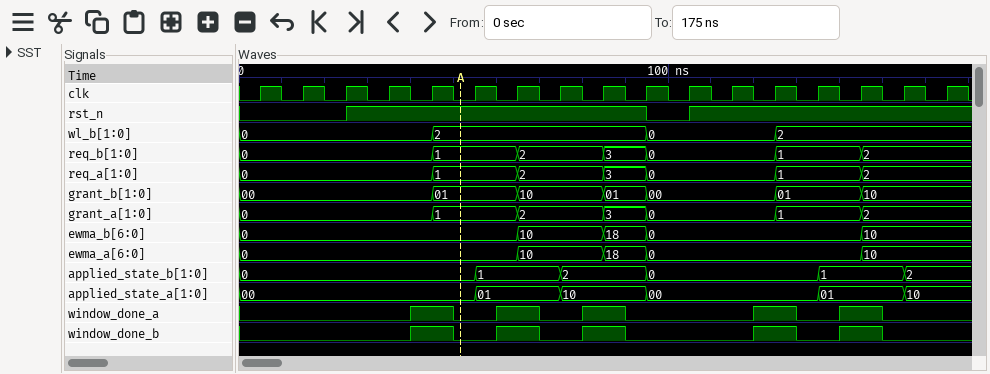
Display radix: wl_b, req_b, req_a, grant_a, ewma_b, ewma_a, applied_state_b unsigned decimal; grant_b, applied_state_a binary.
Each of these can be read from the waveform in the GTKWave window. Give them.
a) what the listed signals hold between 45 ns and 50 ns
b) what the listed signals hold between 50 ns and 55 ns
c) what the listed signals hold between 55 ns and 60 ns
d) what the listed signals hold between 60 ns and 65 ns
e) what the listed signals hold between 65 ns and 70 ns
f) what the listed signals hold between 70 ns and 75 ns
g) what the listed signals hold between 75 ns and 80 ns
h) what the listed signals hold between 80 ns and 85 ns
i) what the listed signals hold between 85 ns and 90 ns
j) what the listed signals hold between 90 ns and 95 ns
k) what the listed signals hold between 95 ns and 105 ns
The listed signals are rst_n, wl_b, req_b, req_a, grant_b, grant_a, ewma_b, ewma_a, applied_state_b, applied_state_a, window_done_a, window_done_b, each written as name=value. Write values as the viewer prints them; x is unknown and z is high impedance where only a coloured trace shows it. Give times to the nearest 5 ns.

rst_n=1, wl_b=2, req_b=1, req_a=1, grant_b=01, grant_a=1, ewma_b=0, ewma_a=0, applied_state_b=0, applied_state_a=00, window_done_a=1, window_done_b=1
rst_n=1, wl_b=2, req_b=1, req_a=1, grant_b=01, grant_a=1, ewma_b=0, ewma_a=0, applied_state_b=0, applied_state_a=00, window_done_a=0, window_done_b=0
rst_n=1, wl_b=2, req_b=1, req_a=1, grant_b=01, grant_a=1, ewma_b=0, ewma_a=0, applied_state_b=1, applied_state_a=01, window_done_a=0, window_done_b=0
rst_n=1, wl_b=2, req_b=1, req_a=1, grant_b=01, grant_a=1, ewma_b=0, ewma_a=0, applied_state_b=1, applied_state_a=01, window_done_a=1, window_done_b=1
rst_n=1, wl_b=2, req_b=2, req_a=2, grant_b=10, grant_a=2, ewma_b=10, ewma_a=10, applied_state_b=1, applied_state_a=01, window_done_a=1, window_done_b=1
rst_n=1, wl_b=2, req_b=2, req_a=2, grant_b=10, grant_a=2, ewma_b=10, ewma_a=10, applied_state_b=1, applied_state_a=01, window_done_a=0, window_done_b=0
rst_n=1, wl_b=2, req_b=2, req_a=2, grant_b=10, grant_a=2, ewma_b=10, ewma_a=10, applied_state_b=2, applied_state_a=10, window_done_a=0, window_done_b=0
rst_n=1, wl_b=2, req_b=2, req_a=2, grant_b=10, grant_a=2, ewma_b=10, ewma_a=10, applied_state_b=2, applied_state_a=10, window_done_a=1, window_done_b=1
rst_n=1, wl_b=2, req_b=3, req_a=3, grant_b=01, grant_a=3, ewma_b=18, ewma_a=18, applied_state_b=2, applied_state_a=10, window_done_a=1, window_done_b=1
rst_n=1, wl_b=2, req_b=3, req_a=3, grant_b=01, grant_a=3, ewma_b=18, ewma_a=18, applied_state_b=2, applied_state_a=10, window_done_a=0, window_done_b=0
rst_n=0, wl_b=0, req_b=0, req_a=0, grant_b=00, grant_a=0, ewma_b=0, ewma_a=0, applied_state_b=0, applied_state_a=00, window_done_a=0, window_done_b=0
